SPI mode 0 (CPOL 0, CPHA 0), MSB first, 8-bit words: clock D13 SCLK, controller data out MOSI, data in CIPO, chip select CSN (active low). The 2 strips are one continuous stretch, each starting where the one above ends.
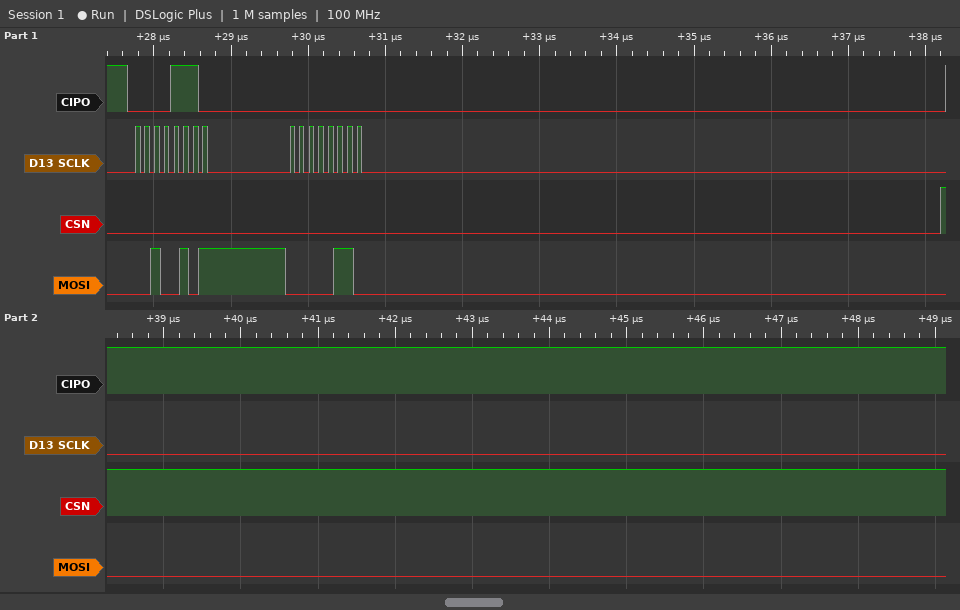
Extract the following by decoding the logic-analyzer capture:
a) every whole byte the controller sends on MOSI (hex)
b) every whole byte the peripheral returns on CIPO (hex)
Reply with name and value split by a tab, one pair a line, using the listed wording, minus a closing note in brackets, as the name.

every whole byte the controller sends on MOSI	25 06
every whole byte the peripheral returns on CIPO	0E 00
